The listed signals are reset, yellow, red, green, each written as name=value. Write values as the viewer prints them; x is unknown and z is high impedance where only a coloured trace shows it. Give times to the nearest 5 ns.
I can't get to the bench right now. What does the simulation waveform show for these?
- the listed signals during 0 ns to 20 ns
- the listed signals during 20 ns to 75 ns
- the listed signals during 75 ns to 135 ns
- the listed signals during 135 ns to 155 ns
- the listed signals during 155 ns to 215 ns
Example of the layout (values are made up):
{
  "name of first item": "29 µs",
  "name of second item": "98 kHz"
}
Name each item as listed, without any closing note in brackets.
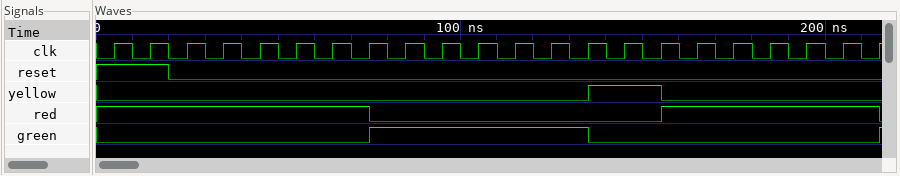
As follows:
{
  "the listed signals during 0 ns to 20 ns": "reset=1, yellow=0, red=1, green=0",
  "the listed signals during 20 ns to 75 ns": "reset=0, yellow=0, red=1, green=0",
  "the listed signals during 75 ns to 135 ns": "reset=0, yellow=0, red=0, green=1",
  "the listed signals during 135 ns to 155 ns": "reset=0, yellow=1, red=0, green=0",
  "the listed signals during 155 ns to 215 ns": "reset=0, yellow=0, red=1, green=0"
}
